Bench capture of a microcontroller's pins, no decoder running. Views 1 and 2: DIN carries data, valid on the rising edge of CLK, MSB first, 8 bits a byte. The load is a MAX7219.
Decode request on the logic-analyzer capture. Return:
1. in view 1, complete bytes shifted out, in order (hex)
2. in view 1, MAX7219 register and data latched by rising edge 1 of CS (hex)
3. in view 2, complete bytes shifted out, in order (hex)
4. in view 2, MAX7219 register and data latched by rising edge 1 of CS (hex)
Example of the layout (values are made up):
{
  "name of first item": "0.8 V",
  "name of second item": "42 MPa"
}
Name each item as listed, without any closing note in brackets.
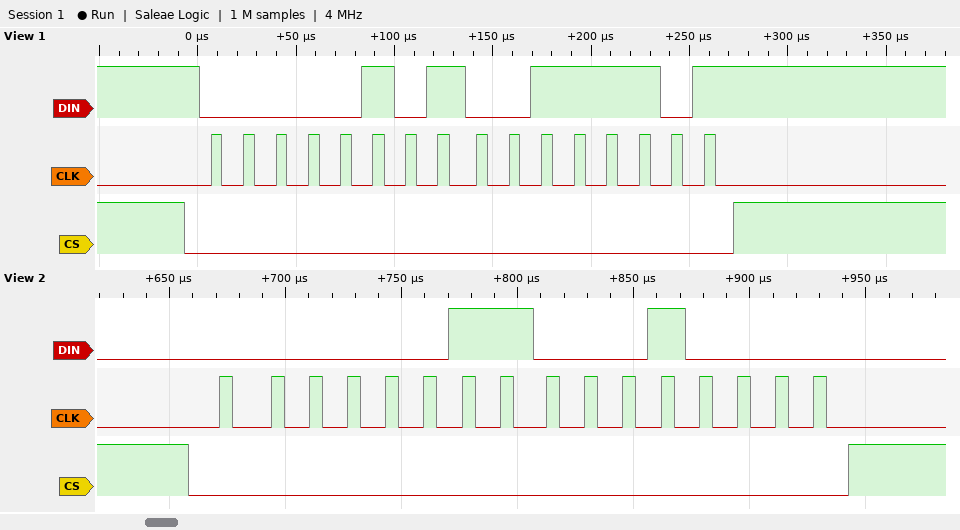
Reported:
{
  "in view 1, complete bytes shifted out, in order": "05 3D",
  "in view 1, MAX7219 register and data latched by rising edge 1 of CS": "register 0x5, data 0x3D",
  "in view 2, complete bytes shifted out, in order": "03 10",
  "in view 2, MAX7219 register and data latched by rising edge 1 of CS": "register 0x3, data 0x10"
}
